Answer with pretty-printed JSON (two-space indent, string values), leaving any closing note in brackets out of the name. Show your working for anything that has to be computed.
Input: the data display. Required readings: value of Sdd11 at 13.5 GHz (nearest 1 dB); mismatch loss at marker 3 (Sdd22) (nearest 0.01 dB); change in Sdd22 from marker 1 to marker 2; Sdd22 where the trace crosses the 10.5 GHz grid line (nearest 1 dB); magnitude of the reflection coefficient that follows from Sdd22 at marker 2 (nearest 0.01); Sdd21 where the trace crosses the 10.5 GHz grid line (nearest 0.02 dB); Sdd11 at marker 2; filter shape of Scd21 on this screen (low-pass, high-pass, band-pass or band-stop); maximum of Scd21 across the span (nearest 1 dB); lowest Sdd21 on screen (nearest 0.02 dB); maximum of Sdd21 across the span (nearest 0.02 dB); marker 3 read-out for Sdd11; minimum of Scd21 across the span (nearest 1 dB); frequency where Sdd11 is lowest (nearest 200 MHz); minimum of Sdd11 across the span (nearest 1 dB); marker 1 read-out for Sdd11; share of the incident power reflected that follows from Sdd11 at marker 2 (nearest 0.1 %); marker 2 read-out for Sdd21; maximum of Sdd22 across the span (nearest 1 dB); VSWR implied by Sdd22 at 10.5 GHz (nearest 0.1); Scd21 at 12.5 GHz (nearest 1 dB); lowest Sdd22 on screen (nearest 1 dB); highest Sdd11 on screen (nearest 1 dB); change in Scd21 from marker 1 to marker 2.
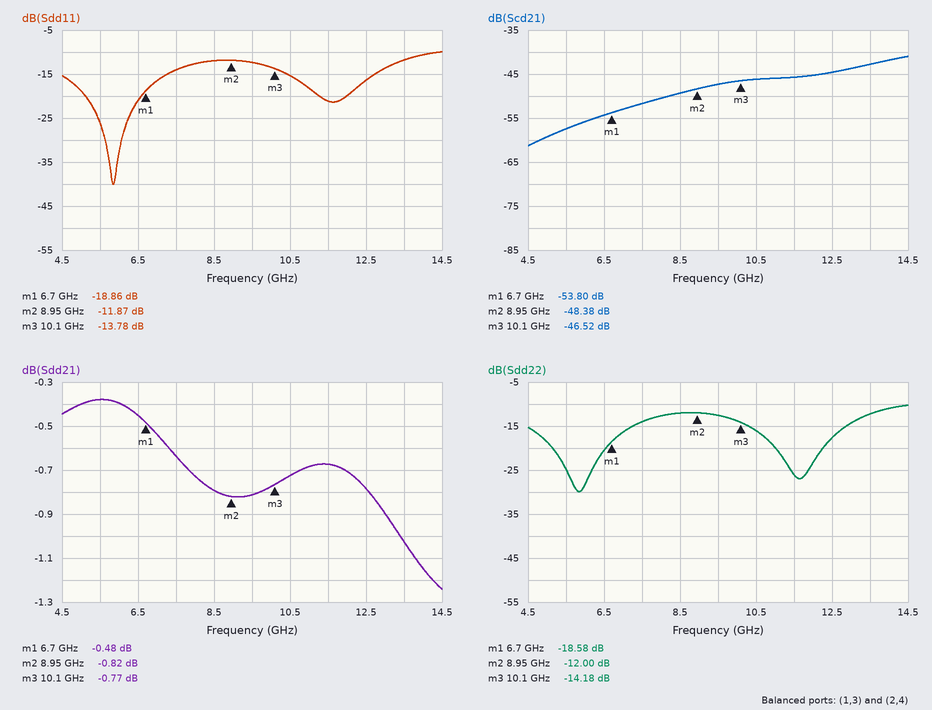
{
  "value of Sdd11 at 13.5 GHz": "-12 dB",
  "mismatch loss at marker 3 (Sdd22)": "−10 log10(1 − 10^(-14.18/10)) ≈ 0.17 dB",
  "change in Sdd22 from marker 1 to marker 2": "-12 − (-18.58) = 6.58 dB",
  "Sdd22 where the trace crosses the 10.5 GHz grid line": "-16 dB",
  "magnitude of the reflection coefficient that follows from Sdd22 at marker 2": "10^(-12/20) ≈ 0.25",
  "Sdd21 where the trace crosses the 10.5 GHz grid line": "-0.72 dB",
  "Sdd11 at marker 2": "-11.87 dB",
  "filter shape of Scd21 on this screen": "high-pass",
  "maximum of Scd21 across the span": "-41 dB",
  "lowest Sdd21 on screen": "-1.24 dB",
  "maximum of Sdd21 across the span": "-0.38 dB",
  "marker 3 read-out for Sdd11": "-13.78 dB",
  "minimum of Scd21 across the span": "-61 dB",
  "frequency where Sdd11 is lowest": "5.8 GHz",
  "minimum of Sdd11 across the span": "-40 dB",
  "marker 1 read-out for Sdd11": "-18.86 dB",
  "share of the incident power reflected that follows from Sdd11 at marker 2": "10^(-11.87/10) ≈ 6.5 %",
  "marker 2 read-out for Sdd21": "-0.82 dB",
  "maximum of Sdd22 across the span": "-10 dB",
  "VSWR implied by Sdd22 at 10.5 GHz": "|Γ| = 10^(-16/20) = 0.1585; VSWR = (1 + 0.1585)/(1 − 0.1585) ≈ 1.4",
  "Scd21 at 12.5 GHz": "-45 dB",
  "lowest Sdd22 on screen": "-30 dB",
  "highest Sdd11 on screen": "-10 dB",
  "change in Scd21 from marker 1 to marker 2": "-48.38 − (-53.8) = 5.42 dB"
}
